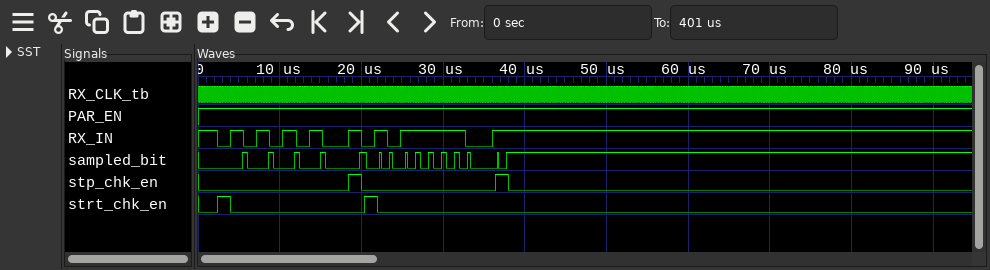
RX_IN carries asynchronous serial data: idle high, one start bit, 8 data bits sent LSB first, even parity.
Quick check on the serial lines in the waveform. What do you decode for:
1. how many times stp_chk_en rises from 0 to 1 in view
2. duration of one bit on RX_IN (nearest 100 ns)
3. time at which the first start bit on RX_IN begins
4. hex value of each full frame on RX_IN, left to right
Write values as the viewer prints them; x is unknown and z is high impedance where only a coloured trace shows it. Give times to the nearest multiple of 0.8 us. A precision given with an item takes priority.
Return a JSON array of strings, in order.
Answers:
["2", "1600 ns", "2.4 us", "55, 7D"]
